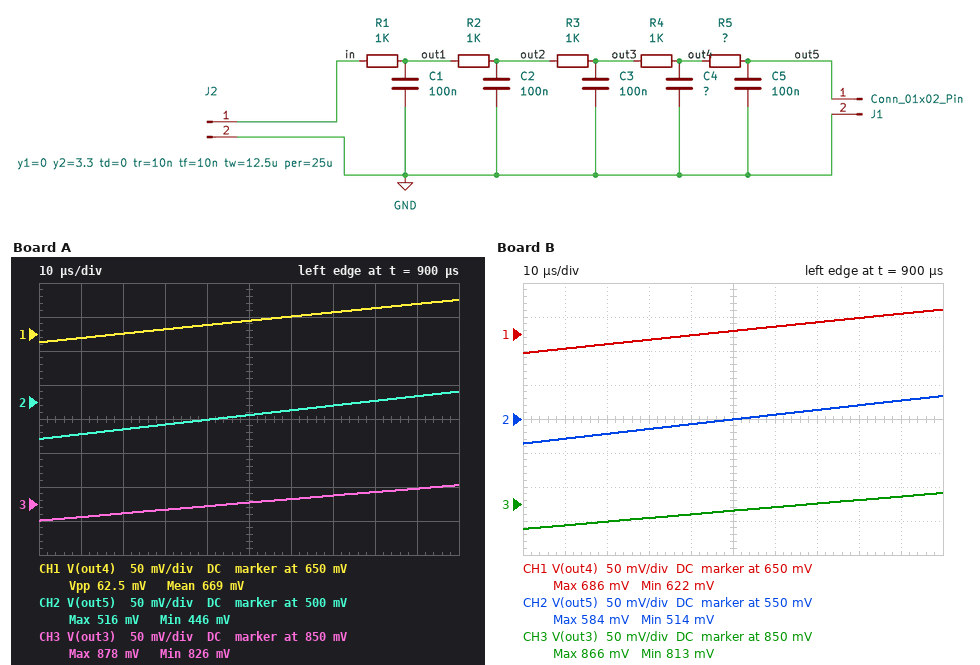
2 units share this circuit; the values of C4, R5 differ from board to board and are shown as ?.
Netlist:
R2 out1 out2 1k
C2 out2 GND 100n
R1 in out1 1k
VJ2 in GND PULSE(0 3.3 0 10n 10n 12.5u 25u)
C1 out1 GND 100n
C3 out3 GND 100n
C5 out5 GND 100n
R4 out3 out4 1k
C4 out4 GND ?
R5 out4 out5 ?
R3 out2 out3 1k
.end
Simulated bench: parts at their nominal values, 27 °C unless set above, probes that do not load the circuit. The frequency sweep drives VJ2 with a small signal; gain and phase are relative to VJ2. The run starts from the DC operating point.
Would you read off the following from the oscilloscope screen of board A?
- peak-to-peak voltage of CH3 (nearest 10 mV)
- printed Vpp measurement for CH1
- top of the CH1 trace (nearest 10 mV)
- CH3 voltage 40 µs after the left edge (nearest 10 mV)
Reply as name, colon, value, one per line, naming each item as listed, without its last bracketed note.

peak-to-peak voltage of CH3: 50 mV
printed Vpp measurement for CH1: 62.5 mV
top of the CH1 trace: 700 mV
CH3 voltage 40 µs after the left edge: 850 mV
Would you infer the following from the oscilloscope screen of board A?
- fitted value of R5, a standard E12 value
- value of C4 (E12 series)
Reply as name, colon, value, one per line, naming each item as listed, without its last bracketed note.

fitted value of R5, a standard E12 value: 2.7 kΩ
value of C4: 180 nF
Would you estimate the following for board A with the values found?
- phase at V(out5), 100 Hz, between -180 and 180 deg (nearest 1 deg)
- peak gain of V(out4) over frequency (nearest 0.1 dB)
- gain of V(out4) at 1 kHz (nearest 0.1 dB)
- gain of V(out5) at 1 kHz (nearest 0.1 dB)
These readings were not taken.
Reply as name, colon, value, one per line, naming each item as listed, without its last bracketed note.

phase at V(out5), 100 Hz, between -180 and 180 deg: -59 deg
peak gain of V(out4) over frequency: 0 dB
gain of V(out4) at 1 kHz: -20.9 dB
gain of V(out5) at 1 kHz: -26.8 dB
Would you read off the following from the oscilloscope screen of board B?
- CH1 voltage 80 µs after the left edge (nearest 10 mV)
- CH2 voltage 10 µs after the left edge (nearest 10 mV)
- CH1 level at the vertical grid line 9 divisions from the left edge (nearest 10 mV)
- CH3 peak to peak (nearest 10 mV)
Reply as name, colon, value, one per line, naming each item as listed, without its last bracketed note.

CH1 voltage 80 µs after the left edge: 670 mV
CH2 voltage 10 µs after the left edge: 520 mV
CH1 level at the vertical grid line 9 divisions from the left edge: 680 mV
CH3 peak to peak: 50 mV
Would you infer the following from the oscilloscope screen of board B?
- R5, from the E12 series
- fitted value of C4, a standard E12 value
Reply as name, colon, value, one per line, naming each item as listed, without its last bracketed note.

R5, from the E12 series: 1.5 kΩ
fitted value of C4, a standard E12 value: 180 nF
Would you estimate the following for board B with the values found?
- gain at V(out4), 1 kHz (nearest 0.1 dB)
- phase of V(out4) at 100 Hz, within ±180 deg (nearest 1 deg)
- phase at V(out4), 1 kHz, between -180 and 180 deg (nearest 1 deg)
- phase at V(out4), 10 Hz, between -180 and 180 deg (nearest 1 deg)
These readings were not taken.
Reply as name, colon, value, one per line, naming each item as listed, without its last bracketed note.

gain at V(out4), 1 kHz: -21.7 dB
phase of V(out4) at 100 Hz, within ±180 deg: -50 deg
phase at V(out4), 1 kHz, between -180 and 180 deg: -140 deg
phase at V(out4), 10 Hz, between -180 and 180 deg: -6 deg
